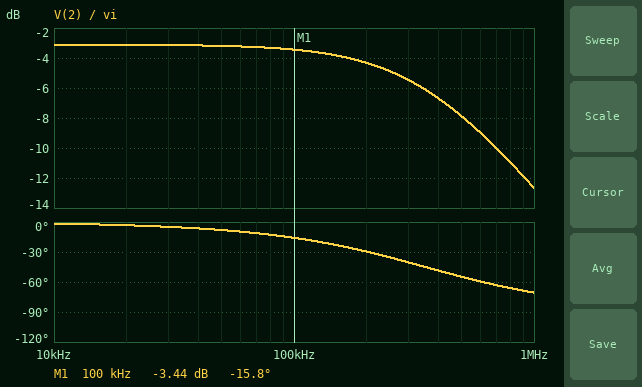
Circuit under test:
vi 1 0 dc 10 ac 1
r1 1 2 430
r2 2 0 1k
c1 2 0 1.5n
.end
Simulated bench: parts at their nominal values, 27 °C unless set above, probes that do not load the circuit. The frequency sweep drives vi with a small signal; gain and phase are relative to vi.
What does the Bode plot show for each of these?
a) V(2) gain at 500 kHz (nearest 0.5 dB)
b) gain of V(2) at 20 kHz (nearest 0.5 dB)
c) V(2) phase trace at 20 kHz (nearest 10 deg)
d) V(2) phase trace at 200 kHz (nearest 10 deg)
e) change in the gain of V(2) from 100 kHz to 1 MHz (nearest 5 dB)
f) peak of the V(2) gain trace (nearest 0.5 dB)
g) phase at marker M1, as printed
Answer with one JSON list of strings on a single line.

["-8.0 dB", "-3.0 dB", "0 deg", "-30 deg", "-10 dB", "-3.0 dB", "-15.8 deg"]
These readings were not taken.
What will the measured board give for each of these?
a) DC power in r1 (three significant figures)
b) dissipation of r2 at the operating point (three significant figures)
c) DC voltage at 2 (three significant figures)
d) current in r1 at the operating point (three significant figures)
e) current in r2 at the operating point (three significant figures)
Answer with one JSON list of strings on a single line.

["21.0 mW", "48.9 mW", "6.99 V", "6.99 mA", "6.99 mA"]
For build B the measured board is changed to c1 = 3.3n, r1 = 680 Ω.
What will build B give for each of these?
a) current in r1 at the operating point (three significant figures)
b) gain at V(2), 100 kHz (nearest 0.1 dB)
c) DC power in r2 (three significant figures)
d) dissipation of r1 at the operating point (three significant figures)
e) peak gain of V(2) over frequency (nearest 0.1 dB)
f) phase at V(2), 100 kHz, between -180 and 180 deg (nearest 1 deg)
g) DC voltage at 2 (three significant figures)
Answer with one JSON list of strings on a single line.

["5.95 mA", "-6.8 dB", "35.4 mW", "24.1 mW", "-4.5 dB", "-40 deg", "5.95 V"]
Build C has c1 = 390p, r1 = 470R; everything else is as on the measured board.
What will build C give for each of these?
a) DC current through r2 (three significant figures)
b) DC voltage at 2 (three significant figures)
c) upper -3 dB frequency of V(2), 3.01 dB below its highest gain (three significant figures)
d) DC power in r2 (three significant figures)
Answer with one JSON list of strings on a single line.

["6.80 mA", "6.80 V", "1.28 MHz", "46.3 mW"]
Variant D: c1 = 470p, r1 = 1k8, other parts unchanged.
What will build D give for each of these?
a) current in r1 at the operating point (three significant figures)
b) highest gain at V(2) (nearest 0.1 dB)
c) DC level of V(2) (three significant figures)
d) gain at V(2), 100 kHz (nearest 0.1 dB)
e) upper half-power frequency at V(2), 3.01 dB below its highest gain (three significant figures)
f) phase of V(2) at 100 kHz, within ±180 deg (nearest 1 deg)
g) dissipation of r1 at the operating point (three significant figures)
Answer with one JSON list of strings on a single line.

["3.57 mA", "-8.9 dB", "3.57 V", "-9.1 dB", "527 kHz", "-11 deg", "23.0 mW"]
